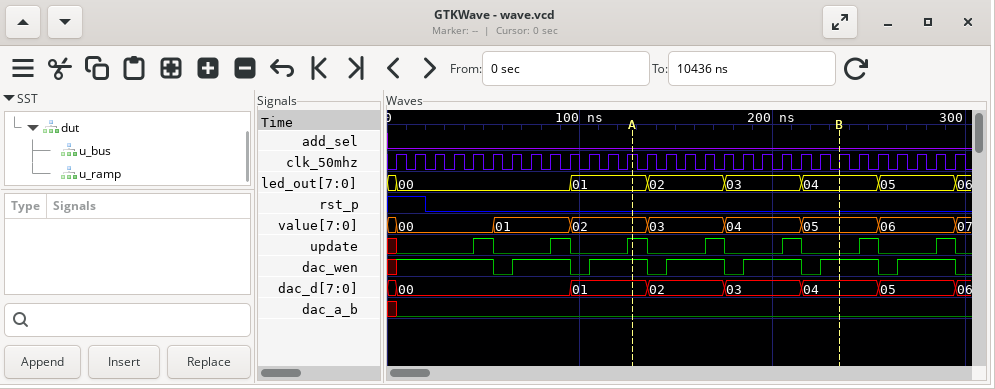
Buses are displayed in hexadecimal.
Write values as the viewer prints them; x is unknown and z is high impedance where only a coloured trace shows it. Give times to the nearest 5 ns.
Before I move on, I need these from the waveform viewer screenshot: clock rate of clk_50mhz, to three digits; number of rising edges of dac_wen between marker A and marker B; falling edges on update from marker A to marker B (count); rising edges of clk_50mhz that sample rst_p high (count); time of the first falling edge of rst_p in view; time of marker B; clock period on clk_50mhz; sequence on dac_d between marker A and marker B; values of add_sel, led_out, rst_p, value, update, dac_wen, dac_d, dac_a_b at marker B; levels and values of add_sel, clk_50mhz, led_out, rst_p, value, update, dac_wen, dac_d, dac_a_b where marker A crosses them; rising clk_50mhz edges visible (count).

100 MHz
3
3
2
20 ns
235 ns
10 ns
01, 02, 03, 04
add_sel=0, led_out=04, rst_p=0, value=05, update=0, dac_wen=1, dac_d=04, dac_a_b=0
add_sel=0, clk_50mhz=1, led_out=01, rst_p=0, value=02, update=1, dac_wen=1, dac_d=01, dac_a_b=0
30
